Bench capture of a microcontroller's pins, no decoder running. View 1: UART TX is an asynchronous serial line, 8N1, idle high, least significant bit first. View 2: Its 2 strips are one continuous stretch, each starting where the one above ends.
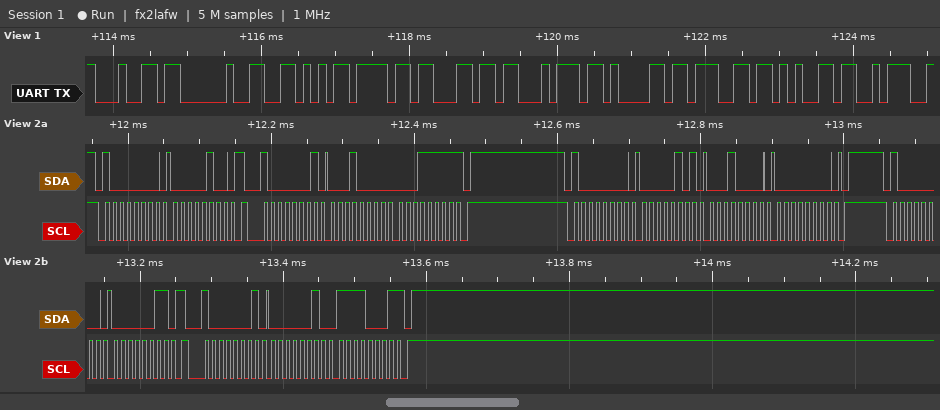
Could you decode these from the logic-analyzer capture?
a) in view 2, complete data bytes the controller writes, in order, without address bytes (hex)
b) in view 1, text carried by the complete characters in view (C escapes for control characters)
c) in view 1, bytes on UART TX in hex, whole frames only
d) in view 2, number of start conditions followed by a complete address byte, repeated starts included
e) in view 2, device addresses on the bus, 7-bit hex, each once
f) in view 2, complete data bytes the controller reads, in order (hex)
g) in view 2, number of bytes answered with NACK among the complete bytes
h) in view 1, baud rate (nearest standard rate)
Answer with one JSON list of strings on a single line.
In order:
["04 05 10 00 03", "\"d Voltage:\"", "64 20 56 6F 6C 74 61 67 65 3A", "5", "0x40", "10 1F 02 F1", "2", "9600 baud"]
